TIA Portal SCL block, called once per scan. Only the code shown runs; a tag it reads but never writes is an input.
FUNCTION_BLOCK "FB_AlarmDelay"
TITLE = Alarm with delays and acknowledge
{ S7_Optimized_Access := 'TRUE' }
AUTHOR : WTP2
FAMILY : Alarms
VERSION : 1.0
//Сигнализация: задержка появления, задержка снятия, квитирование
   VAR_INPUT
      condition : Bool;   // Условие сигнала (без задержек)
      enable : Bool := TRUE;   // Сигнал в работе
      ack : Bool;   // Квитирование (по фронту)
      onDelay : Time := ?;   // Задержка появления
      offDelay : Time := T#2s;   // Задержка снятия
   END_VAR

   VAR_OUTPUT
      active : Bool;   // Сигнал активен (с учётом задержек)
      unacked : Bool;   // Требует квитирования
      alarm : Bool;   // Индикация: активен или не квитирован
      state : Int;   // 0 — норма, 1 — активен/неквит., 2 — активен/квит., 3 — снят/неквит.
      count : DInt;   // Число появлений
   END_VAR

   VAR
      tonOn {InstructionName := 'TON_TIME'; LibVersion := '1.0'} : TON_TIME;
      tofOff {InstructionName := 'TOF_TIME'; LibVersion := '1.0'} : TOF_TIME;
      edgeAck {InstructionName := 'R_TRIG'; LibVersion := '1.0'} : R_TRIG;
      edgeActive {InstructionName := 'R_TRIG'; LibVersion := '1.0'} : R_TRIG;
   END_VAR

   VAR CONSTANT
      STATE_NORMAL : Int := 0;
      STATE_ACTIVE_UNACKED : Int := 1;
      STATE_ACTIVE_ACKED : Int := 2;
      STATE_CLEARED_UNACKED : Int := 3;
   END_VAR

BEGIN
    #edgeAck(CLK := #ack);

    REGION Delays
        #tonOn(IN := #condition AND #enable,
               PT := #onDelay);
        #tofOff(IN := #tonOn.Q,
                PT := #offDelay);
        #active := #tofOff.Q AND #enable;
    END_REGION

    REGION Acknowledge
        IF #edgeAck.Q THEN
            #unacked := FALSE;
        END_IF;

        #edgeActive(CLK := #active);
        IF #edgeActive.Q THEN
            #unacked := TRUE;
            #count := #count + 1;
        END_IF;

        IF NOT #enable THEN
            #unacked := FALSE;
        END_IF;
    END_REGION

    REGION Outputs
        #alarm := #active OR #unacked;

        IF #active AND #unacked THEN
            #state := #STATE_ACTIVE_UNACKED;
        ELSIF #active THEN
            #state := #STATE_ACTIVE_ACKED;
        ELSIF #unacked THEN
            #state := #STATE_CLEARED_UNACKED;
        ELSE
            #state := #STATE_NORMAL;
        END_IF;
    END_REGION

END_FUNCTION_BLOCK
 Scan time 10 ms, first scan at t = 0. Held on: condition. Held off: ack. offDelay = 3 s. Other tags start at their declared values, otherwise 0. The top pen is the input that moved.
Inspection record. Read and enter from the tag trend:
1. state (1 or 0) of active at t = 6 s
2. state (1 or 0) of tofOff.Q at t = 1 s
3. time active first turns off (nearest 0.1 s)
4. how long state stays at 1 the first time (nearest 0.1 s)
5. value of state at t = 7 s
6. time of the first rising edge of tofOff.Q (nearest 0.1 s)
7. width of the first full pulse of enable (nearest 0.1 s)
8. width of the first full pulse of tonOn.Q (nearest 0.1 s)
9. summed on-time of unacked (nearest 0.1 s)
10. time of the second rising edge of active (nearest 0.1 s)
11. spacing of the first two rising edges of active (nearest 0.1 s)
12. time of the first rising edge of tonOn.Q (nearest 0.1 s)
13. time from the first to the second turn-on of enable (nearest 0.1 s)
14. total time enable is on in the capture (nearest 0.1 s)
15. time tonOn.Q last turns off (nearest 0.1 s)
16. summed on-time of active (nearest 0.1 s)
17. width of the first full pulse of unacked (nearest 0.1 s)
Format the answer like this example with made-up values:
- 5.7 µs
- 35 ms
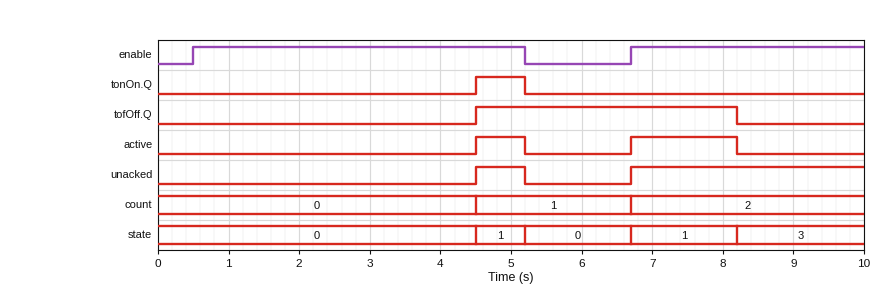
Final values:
- 0
- 0
- 5.2 s
- 0.7 s
- 1
- 4.5 s
- 4.7 s
- 0.7 s
- 4.0 s
- 6.7 s
- 2.2 s
- 4.5 s
- 6.2 s
- 8.0 s
- 5.2 s
- 2.2 s
- 0.7 s
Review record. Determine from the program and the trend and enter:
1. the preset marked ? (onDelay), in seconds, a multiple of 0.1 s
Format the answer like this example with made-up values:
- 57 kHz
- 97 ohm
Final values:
- 4.0 s
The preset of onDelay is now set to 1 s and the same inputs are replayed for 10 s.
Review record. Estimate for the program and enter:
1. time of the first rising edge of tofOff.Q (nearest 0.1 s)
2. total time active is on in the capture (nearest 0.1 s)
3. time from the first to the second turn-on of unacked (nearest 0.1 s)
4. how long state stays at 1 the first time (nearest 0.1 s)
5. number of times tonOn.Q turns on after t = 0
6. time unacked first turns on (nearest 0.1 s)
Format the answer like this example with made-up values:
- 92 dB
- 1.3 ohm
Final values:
- 1.5 s
- 7.0 s
- 5.2 s
- 3.7 s
- 2
- 1.5 s
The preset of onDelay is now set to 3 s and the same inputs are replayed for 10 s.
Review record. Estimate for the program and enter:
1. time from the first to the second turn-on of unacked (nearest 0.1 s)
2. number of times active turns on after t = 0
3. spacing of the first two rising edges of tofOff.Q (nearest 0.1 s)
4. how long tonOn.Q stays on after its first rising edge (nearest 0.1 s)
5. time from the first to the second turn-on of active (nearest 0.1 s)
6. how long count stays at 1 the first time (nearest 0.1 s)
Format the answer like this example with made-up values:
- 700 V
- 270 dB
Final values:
- 3.2 s
- 3
- 6.2 s
- 1.7 s
- 3.2 s
- 3.2 s
